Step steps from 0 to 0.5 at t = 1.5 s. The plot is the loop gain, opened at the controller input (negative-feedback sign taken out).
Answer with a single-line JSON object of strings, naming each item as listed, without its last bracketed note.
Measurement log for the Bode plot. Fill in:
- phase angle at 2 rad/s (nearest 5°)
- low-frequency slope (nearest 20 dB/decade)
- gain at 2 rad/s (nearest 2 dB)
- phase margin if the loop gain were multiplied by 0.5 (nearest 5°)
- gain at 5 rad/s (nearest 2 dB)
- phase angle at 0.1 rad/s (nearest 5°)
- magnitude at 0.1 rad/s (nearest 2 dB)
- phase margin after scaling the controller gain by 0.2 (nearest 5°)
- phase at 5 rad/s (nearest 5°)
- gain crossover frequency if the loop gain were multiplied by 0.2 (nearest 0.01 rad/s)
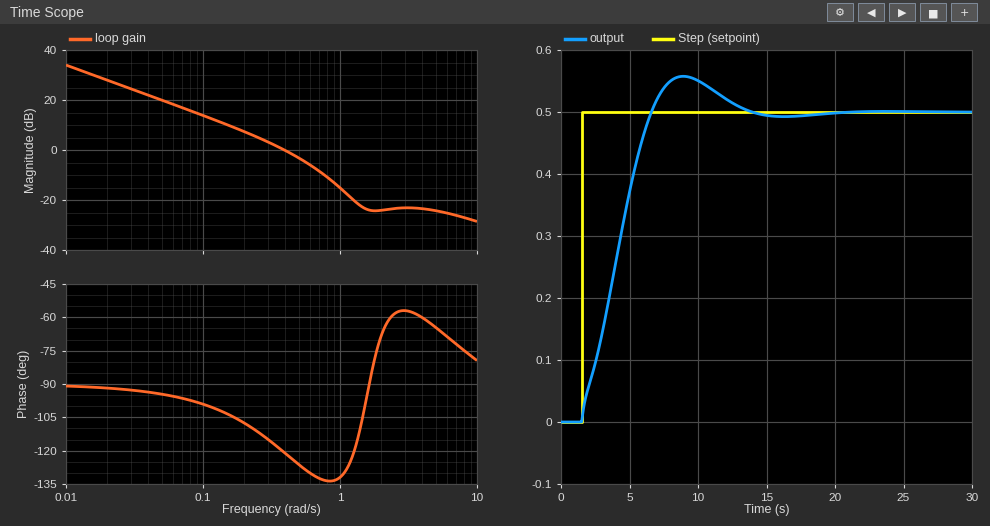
{"phase angle at 2 rad/s": "-70°", "low-frequency slope": "-20 dB/decade", "gain at 2 rad/s": "-24 dB", "phase margin if the loop gain were multiplied by 0.5": "70°", "gain at 5 rad/s": "-24 dB", "phase angle at 0.1 rad/s": "-100°", "magnitude at 0.1 rad/s": "14 dB", "phase margin after scaling the controller gain by 0.2": "80°", "phase at 5 rad/s": "-65°", "gain crossover frequency if the loop gain were multiplied by 0.2": "0.10 rad/s"}
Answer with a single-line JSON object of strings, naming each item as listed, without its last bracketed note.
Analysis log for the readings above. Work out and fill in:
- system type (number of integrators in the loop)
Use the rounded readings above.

{"system type": "1"}
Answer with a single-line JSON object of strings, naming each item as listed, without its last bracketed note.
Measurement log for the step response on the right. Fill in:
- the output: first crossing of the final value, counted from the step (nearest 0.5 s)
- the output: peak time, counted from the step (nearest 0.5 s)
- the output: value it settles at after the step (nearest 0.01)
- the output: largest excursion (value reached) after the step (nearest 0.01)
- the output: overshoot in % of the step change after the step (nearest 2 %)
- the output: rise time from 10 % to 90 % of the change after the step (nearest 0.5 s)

{"the output: first crossing of the final value, counted from the step": "5.0 s", "the output: peak time, counted from the step": "7.5 s", "the output: value it settles at after the step": "0.50", "the output: largest excursion (value reached) after the step": "0.56", "the output: overshoot in % of the step change after the step": "12 %", "the output: rise time from 10 % to 90 % of the change after the step": "4.0 s"}
